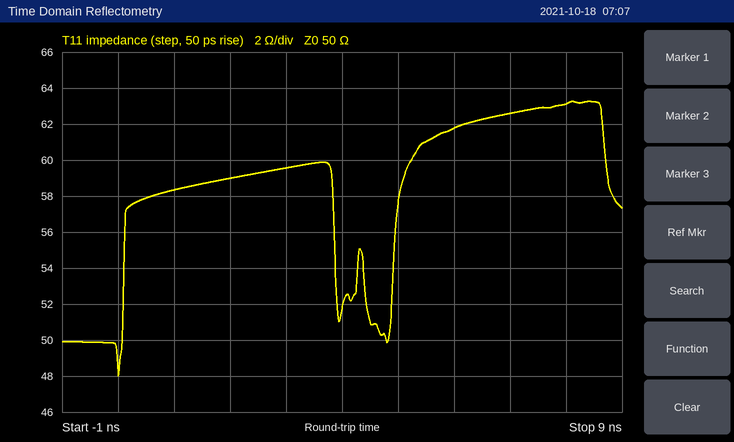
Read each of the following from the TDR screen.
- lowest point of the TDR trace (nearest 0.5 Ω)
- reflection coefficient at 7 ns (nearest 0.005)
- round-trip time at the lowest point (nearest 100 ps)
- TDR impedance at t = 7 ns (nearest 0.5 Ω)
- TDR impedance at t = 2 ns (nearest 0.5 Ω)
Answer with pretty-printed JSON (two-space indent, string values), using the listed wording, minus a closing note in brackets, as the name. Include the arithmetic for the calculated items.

{
  "lowest point of the TDR trace": "48.0 Ω",
  "reflection coefficient at 7 ns": "(62.5 − 50)/(62.5 + 50) ≈ +0.111, so +0.110 to the nearest 0.005",
  "round-trip time at the lowest point": "0.0 ns",
  "TDR impedance at t = 7 ns": "62.5 Ω",
  "TDR impedance at t = 2 ns": "59.0 Ω"
}
